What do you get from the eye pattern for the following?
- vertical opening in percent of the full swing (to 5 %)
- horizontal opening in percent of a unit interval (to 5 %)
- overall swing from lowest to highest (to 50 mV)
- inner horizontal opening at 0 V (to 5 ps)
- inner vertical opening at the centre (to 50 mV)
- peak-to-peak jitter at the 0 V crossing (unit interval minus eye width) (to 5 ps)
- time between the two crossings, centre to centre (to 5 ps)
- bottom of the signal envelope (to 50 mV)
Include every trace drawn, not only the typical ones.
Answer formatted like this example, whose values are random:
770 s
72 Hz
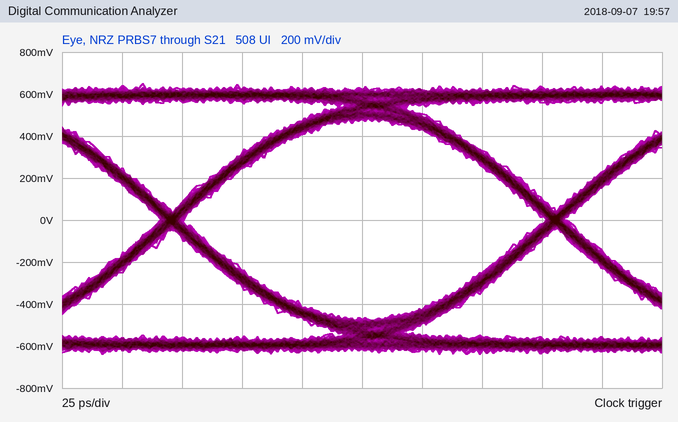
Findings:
75 %
95 %
1.30 V
150 ps
950 mV
10 ps
160 ps
-650 mV
